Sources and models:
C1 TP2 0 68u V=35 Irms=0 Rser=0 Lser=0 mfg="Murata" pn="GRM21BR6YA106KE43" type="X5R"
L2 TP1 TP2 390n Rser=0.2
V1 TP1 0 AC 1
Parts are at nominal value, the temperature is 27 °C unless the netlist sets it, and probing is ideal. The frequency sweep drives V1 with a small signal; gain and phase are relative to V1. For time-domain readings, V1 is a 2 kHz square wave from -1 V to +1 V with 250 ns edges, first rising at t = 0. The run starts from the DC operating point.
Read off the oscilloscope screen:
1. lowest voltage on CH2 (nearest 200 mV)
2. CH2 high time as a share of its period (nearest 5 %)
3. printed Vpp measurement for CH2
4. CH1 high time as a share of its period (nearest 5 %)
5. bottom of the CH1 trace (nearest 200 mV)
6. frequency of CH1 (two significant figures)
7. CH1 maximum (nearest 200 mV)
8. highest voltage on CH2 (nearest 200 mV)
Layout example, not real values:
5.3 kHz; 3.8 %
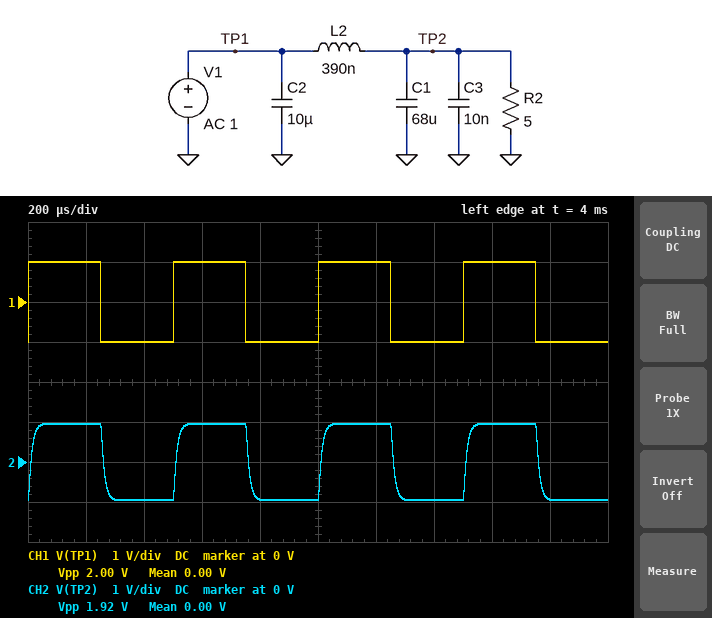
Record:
-1.0 V; 50 %; 1.92 V; 50 %; -1.0 V; 2.0 kHz; 1.0 V; 1.0 V
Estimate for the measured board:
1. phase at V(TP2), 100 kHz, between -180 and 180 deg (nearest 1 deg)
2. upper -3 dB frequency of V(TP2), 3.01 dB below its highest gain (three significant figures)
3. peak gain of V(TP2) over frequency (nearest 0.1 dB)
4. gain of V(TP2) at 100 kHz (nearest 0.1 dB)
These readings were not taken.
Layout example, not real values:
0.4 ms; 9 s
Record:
-138 deg; 14.1 kHz; -0.3 dB; -22.1 dB
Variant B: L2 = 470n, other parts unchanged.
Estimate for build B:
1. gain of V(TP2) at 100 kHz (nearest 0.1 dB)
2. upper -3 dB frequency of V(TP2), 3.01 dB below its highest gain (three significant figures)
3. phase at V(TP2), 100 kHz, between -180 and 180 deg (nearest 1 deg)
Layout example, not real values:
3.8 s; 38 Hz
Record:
-23.2 dB; 14.5 kHz; -143 deg
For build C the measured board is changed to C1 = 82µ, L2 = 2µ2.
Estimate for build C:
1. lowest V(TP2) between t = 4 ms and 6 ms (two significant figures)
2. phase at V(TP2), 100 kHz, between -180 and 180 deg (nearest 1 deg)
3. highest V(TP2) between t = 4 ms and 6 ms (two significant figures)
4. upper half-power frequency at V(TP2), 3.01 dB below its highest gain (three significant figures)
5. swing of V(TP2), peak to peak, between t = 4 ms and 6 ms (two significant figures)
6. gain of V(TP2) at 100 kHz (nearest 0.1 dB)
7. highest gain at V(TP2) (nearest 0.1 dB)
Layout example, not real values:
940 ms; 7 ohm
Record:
-1.1 V; -171 deg; 1.1 V; 13.3 kHz; 2.3 V; -37.0 dB; -0.1 dB
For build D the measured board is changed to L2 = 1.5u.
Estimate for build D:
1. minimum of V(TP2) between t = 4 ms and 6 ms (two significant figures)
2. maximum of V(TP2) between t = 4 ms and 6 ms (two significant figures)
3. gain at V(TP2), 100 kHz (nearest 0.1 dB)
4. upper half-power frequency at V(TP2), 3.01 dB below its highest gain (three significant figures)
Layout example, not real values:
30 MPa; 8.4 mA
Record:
-1.1 V; 1.1 V; -32.1 dB; 16.7 kHz
